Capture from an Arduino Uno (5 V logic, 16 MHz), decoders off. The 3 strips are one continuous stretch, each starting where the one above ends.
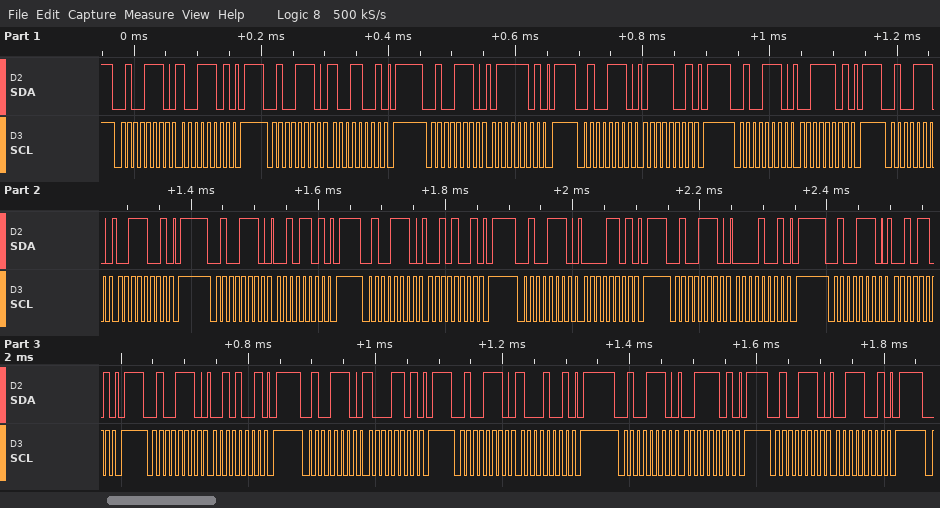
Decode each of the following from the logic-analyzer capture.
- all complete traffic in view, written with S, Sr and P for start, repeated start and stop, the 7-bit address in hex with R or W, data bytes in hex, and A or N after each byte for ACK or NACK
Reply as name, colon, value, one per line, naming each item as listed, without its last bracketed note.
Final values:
all complete traffic in view, written with S, Sr and P for start, repeated start and stop, the 7-bit address in hex with R or W, data bytes in hex, and A or N after each byte for ACK or NACK: S 27W A 9D A P S 27W A 99 A P S 27W A 7D A P S 27W A 79 A P S 27W A 3D A P S 27W A 39 A P S 27W A 2D A P S 27W A 29 A P S 27W A 0D A P S 27W A 09 A P S 27W A 2D A P S 27W A 29 A P S 27W A 8D A P S 27W A 89 A P S 27W A 3D A P S 27W A 39 A P
